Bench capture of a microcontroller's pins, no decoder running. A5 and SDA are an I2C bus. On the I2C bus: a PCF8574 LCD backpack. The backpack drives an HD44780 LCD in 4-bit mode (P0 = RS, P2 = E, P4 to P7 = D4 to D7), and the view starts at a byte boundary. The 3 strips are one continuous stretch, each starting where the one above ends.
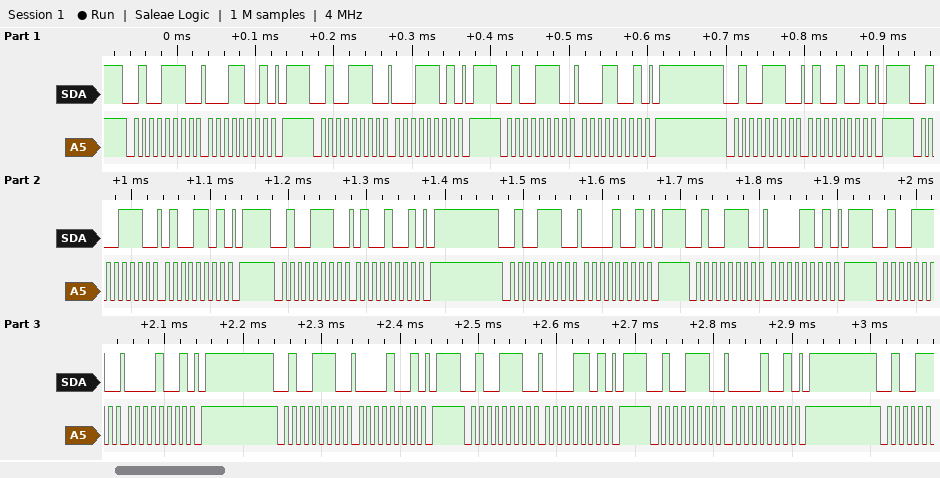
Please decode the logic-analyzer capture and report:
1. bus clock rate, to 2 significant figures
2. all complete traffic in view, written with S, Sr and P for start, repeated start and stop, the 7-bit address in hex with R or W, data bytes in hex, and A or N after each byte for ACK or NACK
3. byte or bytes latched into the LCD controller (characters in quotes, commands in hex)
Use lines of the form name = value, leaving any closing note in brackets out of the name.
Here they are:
bus clock rate, to 2 significant figures = 100 kHz
all complete traffic in view, written with S, Sr and P for start, repeated start and stop, the 7-bit address in hex with R or W, data bytes in hex, and A or N after each byte for ACK or NACK = S 27W A 19 A P S 27W A 1D A P S 27W A 19 A P S 27W A 49 A P S 27W A 4D A P S 27W A 49 A P S 27W A 09 A P S 27W A 0D A P S 27W A 09 A P S 27W A 09 A P S 27W A 0D A P S 27W A 09 A P
byte or bytes latched into the LCD controller = data 0x14 data 0x00
